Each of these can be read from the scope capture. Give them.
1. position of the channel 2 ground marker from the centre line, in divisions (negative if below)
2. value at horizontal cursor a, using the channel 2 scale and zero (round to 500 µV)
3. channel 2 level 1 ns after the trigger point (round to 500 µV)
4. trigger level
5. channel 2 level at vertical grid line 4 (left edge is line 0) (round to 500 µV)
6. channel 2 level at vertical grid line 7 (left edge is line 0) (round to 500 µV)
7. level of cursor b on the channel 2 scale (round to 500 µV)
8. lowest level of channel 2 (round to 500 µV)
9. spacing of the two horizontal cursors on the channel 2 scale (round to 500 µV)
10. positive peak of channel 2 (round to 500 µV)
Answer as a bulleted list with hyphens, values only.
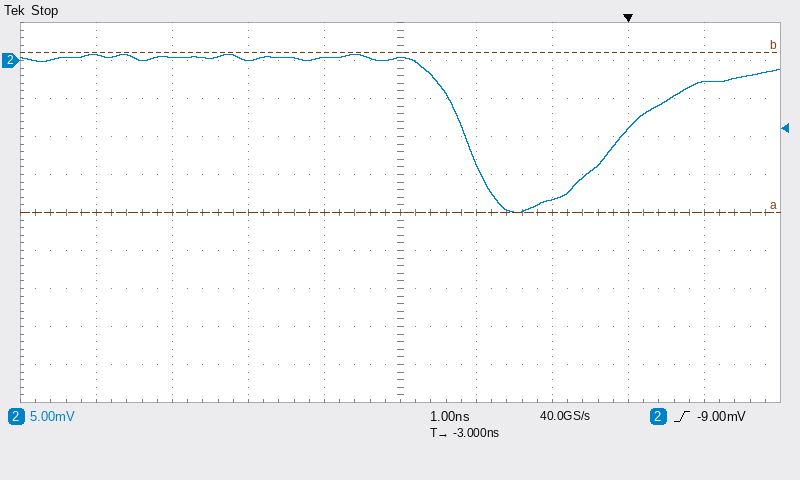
- +4.0 div
- -20.0 mV
- -3.0 mV
- -9.00 mV
- 500 µV
- -18.5 mV
- 1.0 mV
- -20.0 mV
- 21.0 mV
- 1.0 mV
